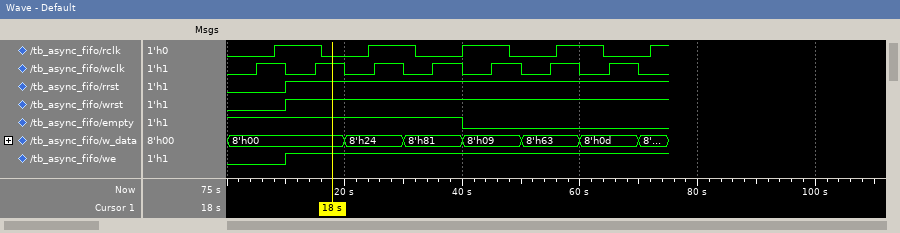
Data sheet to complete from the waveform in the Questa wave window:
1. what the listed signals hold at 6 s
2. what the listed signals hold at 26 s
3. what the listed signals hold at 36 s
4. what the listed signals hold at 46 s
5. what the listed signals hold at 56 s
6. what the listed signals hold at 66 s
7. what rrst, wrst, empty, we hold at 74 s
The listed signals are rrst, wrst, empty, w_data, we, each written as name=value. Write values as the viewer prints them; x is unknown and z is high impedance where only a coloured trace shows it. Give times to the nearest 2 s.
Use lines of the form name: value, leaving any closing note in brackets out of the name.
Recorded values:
what the listed signals hold at 6 s: rrst=0, wrst=0, empty=1, w_data=8'h00, we=0
what the listed signals hold at 26 s: rrst=1, wrst=1, empty=1, w_data=8'h24, we=1
what the listed signals hold at 36 s: rrst=1, wrst=1, empty=1, w_data=8'h81, we=1
what the listed signals hold at 46 s: rrst=1, wrst=1, empty=0, w_data=8'h09, we=1
what the listed signals hold at 56 s: rrst=1, wrst=1, empty=0, w_data=8'h63, we=1
what the listed signals hold at 66 s: rrst=1, wrst=1, empty=0, w_data=8'h0d, we=1
what rrst, wrst, empty, we hold at 74 s: rrst=1, wrst=1, empty=0, we=1
